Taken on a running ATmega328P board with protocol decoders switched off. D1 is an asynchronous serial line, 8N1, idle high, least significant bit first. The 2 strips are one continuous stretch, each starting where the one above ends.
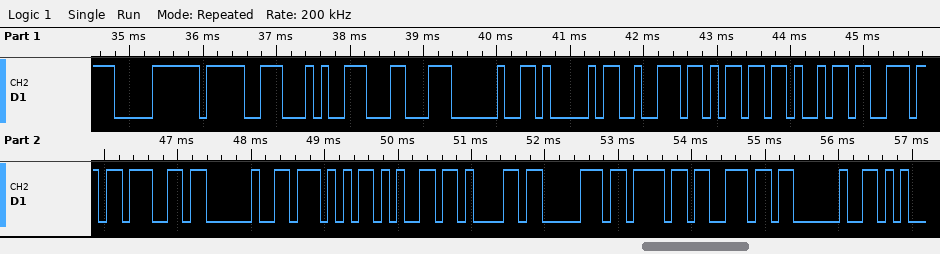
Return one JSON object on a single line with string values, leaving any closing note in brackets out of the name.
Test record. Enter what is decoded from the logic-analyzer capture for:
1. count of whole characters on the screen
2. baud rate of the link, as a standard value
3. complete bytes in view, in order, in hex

{"count of whole characters on the screen": "19", "baud rate of the link, as a standard value": "9600 baud", "complete bytes in view, in order, in hex": "F0 9F 94 8C 20 41 72 6D 69 6E 67 20 57 65 61 70 6F 6E 20"}
